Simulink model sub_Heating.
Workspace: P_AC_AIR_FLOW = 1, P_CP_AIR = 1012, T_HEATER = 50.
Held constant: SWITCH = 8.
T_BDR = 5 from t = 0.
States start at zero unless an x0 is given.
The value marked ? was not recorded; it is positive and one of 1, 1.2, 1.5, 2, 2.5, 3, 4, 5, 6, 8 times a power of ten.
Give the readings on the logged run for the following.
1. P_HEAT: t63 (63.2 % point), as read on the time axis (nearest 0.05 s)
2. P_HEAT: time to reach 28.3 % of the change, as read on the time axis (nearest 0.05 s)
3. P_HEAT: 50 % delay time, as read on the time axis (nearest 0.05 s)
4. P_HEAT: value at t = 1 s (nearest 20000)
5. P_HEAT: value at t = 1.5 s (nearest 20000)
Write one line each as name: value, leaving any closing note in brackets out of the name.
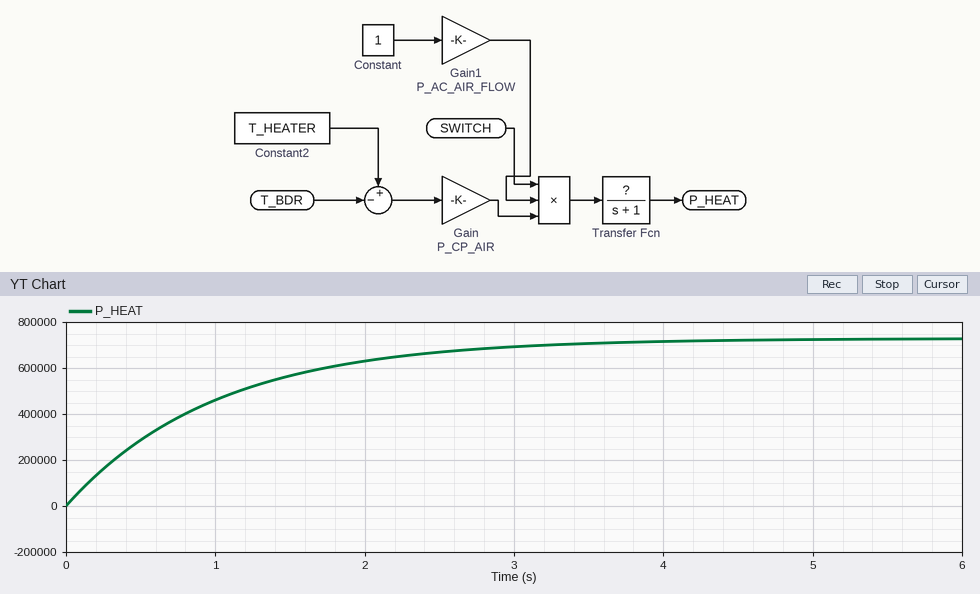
P_HEAT: t63 (63.2 % point), as read on the time axis: 1.00 s
P_HEAT: time to reach 28.3 % of the change, as read on the time axis: 0.35 s
P_HEAT: 50 % delay time, as read on the time axis: 0.70 s
P_HEAT: value at t = 1 s: 460000
P_HEAT: value at t = 1.5 s: 560000
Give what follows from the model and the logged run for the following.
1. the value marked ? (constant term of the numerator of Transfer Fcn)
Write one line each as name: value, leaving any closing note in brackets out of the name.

the value marked ?: 2
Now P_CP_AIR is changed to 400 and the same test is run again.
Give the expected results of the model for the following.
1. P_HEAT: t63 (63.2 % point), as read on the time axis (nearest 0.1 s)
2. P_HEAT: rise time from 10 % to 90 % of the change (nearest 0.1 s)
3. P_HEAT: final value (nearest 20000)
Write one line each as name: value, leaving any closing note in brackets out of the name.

P_HEAT: t63 (63.2 % point), as read on the time axis: 1.0 s
P_HEAT: rise time from 10 % to 90 % of the change: 2.2 s
P_HEAT: final value: 280000
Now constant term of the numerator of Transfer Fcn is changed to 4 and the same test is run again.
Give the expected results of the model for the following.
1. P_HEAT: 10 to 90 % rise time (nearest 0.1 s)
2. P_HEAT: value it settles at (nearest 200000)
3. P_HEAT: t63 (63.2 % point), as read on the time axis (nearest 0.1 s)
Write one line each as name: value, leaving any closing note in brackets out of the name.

P_HEAT: 10 to 90 % rise time: 2.2 s
P_HEAT: value it settles at: 1400000
P_HEAT: t63 (63.2 % point), as read on the time axis: 1.0 s
